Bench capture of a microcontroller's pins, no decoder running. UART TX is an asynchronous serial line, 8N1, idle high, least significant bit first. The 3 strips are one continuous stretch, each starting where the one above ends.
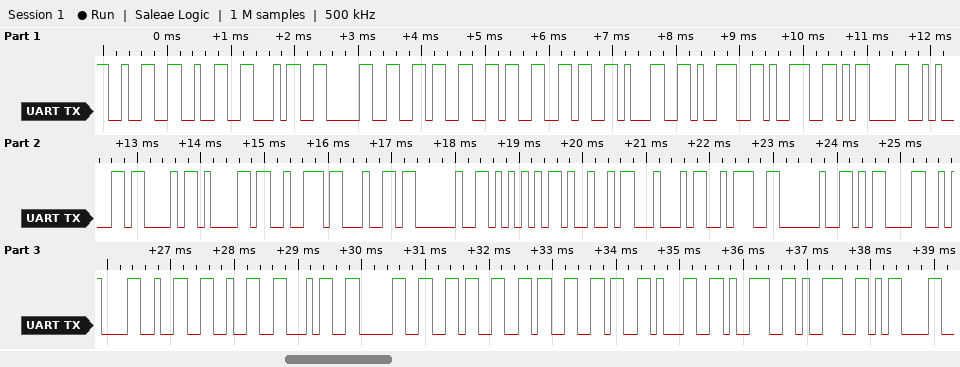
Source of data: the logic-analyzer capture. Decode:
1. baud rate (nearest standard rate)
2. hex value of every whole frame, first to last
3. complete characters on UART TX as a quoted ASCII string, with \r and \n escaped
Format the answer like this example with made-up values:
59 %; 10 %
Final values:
9600 baud; 0x32 0x32 0x34 0x30 0x36 0x36 0x36 0x31 0x39 0x39 0x0D 0x0A 0x43 0x61 0x72 0x64 0x20 0x55 0x49 0x44 0x3A 0x20 0x0D 0x0A 0x32 0x32 0x34 0x30 0x36 0x36 0x36 0x31 0x39 0x39 0x0D; "2240666199\r\nCard UID: \r\n2240666199\r"
